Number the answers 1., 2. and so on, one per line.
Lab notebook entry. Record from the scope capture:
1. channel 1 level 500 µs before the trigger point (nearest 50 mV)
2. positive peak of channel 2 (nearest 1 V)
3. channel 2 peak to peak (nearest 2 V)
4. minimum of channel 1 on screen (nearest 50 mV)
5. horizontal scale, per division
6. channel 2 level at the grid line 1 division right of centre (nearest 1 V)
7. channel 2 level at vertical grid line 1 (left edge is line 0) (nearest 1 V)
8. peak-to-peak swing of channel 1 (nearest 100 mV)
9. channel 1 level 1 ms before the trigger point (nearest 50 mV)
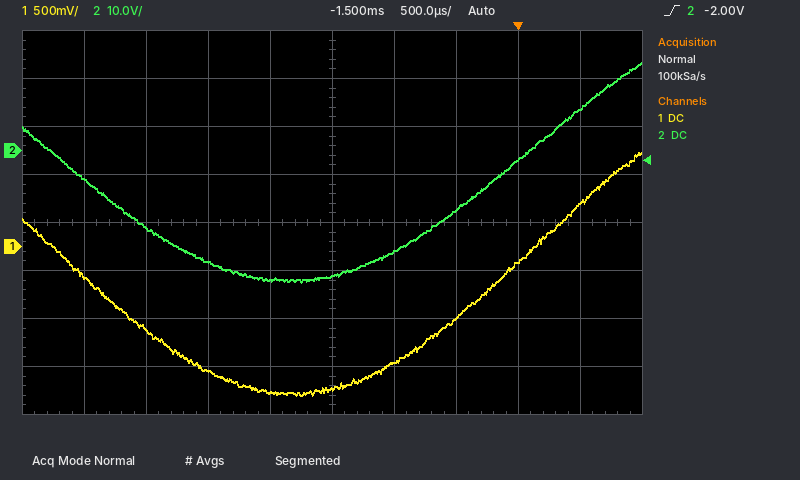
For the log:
1. -750 mV
2. 18 V
3. 46 V
4. -1.55 V
5. 500 µs
6. -21 V
7. -6 V
8. 2.50 V
9. -1.20 V
